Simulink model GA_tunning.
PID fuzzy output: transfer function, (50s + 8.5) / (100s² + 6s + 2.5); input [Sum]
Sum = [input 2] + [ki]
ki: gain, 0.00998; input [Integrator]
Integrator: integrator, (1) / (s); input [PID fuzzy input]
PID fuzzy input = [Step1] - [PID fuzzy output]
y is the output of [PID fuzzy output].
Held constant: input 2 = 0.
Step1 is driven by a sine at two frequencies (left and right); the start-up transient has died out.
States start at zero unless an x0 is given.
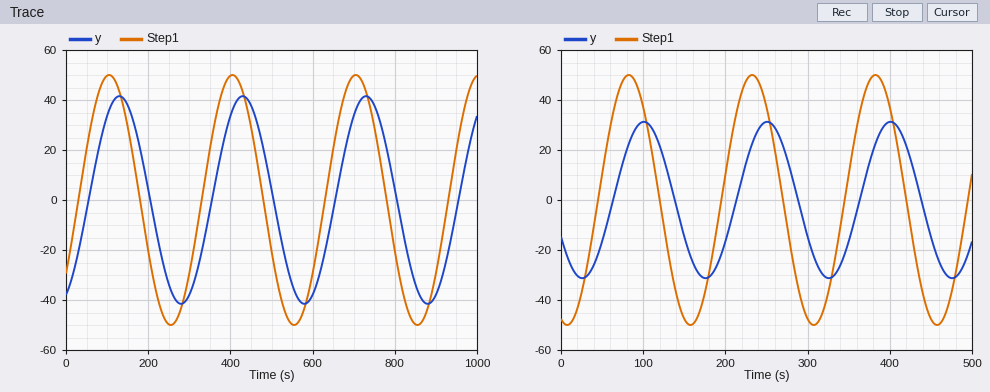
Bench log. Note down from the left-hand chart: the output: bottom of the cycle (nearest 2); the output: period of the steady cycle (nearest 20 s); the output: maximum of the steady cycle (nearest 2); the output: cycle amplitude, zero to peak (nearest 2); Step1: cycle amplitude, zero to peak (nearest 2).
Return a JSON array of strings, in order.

["-42", "300 s", "42", "42", "50"]
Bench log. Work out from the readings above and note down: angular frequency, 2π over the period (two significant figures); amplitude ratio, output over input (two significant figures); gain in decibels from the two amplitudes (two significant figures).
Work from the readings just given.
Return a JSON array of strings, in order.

["0.021 rad/s", "0.84", "-1.5 dB"]
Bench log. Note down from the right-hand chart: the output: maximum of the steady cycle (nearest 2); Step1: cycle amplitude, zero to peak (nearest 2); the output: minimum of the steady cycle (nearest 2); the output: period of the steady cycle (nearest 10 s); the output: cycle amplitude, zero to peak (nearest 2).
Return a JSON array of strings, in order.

["32", "50", "-32", "150 s", "32"]
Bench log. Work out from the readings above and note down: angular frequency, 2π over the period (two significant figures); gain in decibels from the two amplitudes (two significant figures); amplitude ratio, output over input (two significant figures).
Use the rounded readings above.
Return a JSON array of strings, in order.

["0.042 rad/s", "-3.9 dB", "0.64"]
